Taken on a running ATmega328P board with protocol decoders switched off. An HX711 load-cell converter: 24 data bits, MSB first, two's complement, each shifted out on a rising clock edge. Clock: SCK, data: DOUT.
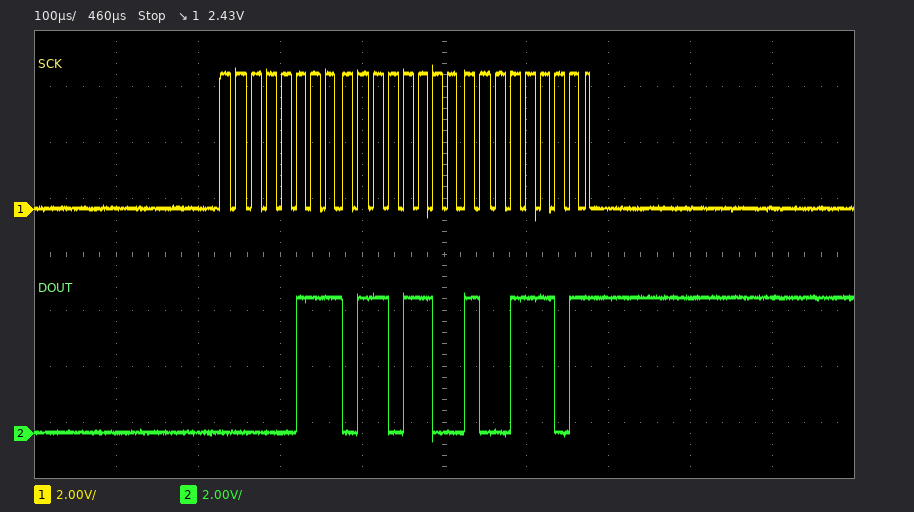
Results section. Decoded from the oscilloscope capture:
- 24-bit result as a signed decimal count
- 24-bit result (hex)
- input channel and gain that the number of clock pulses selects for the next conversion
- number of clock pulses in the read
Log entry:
486557
0x076C9D
channel A, gain 128
25
